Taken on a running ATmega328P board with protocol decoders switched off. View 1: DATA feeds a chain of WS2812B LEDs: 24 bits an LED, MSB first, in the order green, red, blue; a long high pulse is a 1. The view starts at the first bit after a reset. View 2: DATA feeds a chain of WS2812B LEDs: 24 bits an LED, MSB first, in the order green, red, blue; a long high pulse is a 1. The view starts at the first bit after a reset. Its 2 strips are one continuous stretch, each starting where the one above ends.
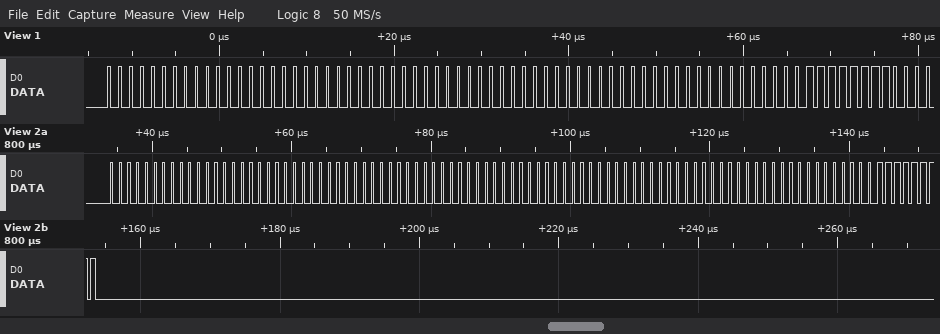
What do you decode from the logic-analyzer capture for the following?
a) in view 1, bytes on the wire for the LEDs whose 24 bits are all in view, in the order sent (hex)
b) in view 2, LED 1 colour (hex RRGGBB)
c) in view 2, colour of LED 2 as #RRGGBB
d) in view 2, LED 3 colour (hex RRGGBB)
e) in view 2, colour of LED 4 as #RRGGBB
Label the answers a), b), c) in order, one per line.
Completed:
a) 00 00 00 00 00 00 00 00 FF
b) #000000
c) #000000
d) #000000
e) #0000FF
